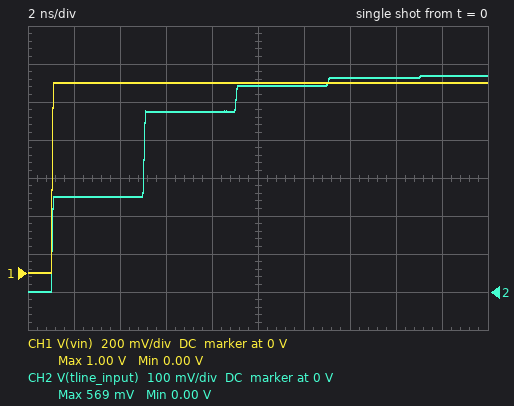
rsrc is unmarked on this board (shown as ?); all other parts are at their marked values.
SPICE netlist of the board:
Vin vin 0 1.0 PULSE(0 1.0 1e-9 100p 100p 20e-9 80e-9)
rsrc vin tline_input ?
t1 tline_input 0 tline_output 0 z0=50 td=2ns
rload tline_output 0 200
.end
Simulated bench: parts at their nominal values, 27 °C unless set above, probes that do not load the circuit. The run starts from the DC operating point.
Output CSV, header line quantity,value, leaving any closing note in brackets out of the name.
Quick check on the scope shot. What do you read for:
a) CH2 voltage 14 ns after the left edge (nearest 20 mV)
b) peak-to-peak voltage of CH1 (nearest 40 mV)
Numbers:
quantity,value
CH2 voltage 14 ns after the left edge,560 mV
peak-to-peak voltage of CH1,1.00 V
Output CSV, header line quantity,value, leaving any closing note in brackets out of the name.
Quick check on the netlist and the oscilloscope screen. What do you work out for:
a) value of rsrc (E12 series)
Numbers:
quantity,value
value of rsrc,150 Ω
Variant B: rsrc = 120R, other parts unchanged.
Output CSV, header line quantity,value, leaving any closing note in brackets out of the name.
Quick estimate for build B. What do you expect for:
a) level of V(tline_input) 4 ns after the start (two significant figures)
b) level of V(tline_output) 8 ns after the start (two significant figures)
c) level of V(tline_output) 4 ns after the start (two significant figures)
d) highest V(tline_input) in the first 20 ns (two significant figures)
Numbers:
quantity,value
level of V(tline_input) 4 ns after the start,290 mV
level of V(tline_output) 8 ns after the start,590 mV
level of V(tline_output) 4 ns after the start,470 mV
highest V(tline_input) in the first 20 ns,620 mV
